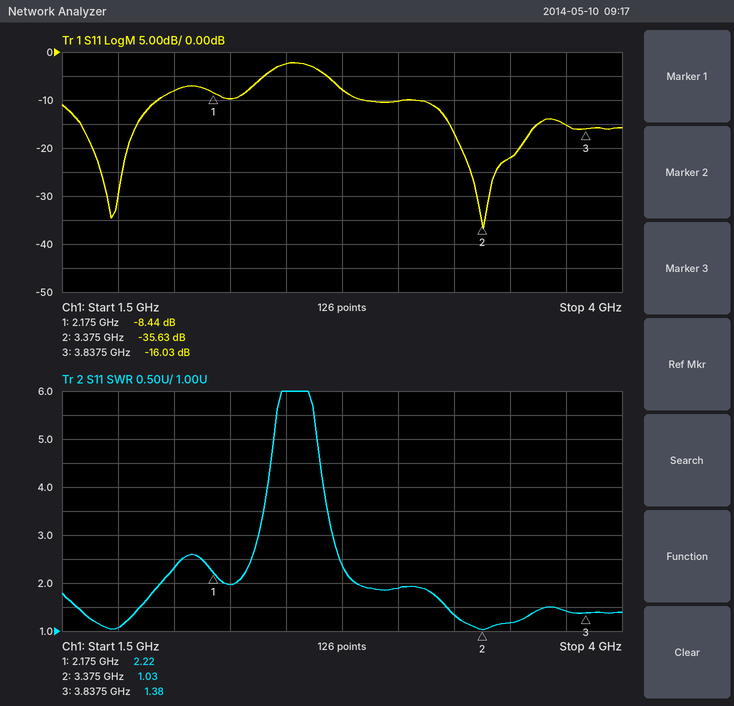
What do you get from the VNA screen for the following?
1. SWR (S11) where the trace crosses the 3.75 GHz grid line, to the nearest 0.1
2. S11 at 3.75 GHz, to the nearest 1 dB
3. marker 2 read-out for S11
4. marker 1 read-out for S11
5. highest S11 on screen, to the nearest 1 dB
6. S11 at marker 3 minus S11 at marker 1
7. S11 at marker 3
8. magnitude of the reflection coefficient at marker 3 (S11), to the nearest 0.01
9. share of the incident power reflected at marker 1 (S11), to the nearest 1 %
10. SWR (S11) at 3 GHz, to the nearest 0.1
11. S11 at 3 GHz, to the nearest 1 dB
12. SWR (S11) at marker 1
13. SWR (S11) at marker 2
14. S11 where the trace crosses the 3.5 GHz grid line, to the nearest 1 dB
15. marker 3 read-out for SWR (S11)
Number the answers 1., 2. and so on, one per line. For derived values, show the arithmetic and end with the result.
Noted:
1. 1.4
2. -15 dB
3. -35.63 dB
4. -8.44 dB
5. -2 dB
6. -16.03 − (-8.44) = -7.59 dB
7. -16.03 dB
8. 10^(-16.03/20) ≈ 0.16
9. 10^(-8.44/10) ≈ 14 %
10. 1.9
11. -10 dB
12. 2.22
13. 1.03
14. -22 dB
15. 1.38
